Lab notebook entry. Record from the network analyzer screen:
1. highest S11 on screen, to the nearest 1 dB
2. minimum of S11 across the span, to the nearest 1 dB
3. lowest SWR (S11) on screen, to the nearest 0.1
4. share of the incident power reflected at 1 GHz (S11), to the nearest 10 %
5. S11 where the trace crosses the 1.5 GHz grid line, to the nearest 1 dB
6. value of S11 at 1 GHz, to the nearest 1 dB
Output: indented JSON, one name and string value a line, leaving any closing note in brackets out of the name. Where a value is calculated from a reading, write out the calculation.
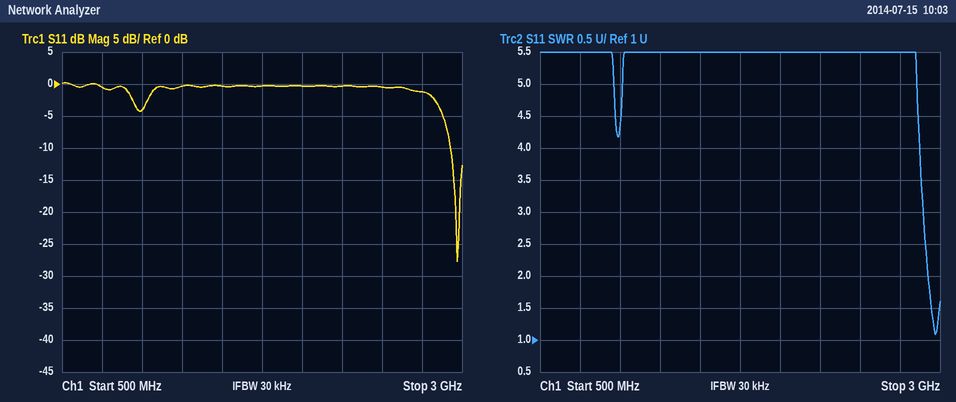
{
  "highest S11 on screen, to the nearest 1 dB": "0 dB",
  "minimum of S11 across the span, to the nearest 1 dB": "-28 dB",
  "lowest SWR (S11) on screen, to the nearest 0.1": "1.1",
  "share of the incident power reflected at 1 GHz (S11), to the nearest 10 %": "10^(-4/10) ≈ 40 %",
  "S11 where the trace crosses the 1.5 GHz grid line, to the nearest 1 dB": "0 dB",
  "value of S11 at 1 GHz, to the nearest 1 dB": "-4 dB"
}
